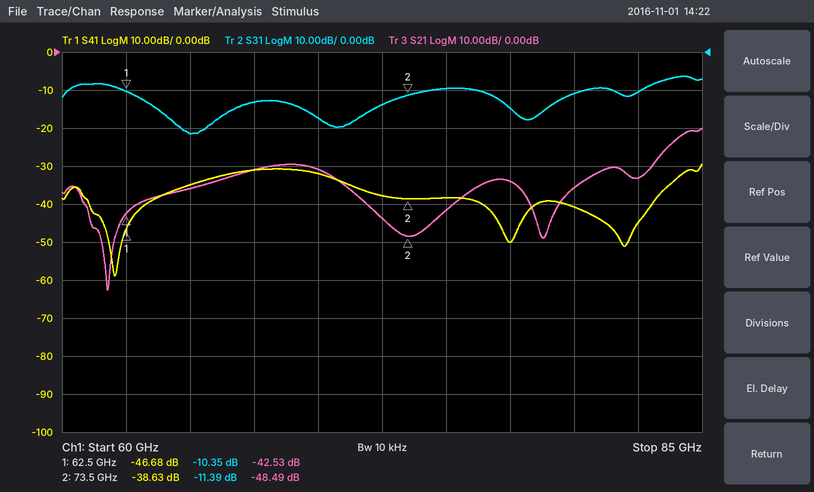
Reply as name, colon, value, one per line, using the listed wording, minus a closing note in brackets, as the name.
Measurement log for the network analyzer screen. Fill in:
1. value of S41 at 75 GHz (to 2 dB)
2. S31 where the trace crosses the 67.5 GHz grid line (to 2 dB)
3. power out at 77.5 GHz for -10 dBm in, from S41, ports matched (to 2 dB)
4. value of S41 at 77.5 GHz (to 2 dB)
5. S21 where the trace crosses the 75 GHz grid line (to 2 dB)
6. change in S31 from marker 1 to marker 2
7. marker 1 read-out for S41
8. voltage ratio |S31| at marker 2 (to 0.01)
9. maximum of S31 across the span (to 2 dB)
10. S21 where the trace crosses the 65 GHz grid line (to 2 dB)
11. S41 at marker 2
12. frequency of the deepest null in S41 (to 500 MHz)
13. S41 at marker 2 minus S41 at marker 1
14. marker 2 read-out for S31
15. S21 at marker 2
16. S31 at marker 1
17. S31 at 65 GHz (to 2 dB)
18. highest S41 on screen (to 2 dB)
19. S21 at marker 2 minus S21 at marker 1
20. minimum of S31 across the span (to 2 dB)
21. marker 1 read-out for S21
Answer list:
value of S41 at 75 GHz: -38 dB
S31 where the trace crosses the 67.5 GHz grid line: -14 dB
power out at 77.5 GHz for -10 dBm in, from S41, ports matched: -60 dBm
value of S41 at 77.5 GHz: -50 dB
S21 where the trace crosses the 75 GHz grid line: -42 dB
change in S31 from marker 1 to marker 2: -1.04 dB
marker 1 read-out for S41: -46.68 dB
voltage ratio |S31| at marker 2: 0.27
maximum of S31 across the span: -6 dB
S21 where the trace crosses the 65 GHz grid line: -36 dB
S41 at marker 2: -38.63 dB
frequency of the deepest null in S41: 62.0 GHz
S41 at marker 2 minus S41 at marker 1: 8.05 dB
marker 2 read-out for S31: -11.39 dB
S21 at marker 2: -48.49 dB
S31 at marker 1: -10.35 dB
S31 at 65 GHz: -22 dB
highest S41 on screen: -30 dB
S21 at marker 2 minus S21 at marker 1: -5.96 dB
minimum of S31 across the span: -22 dB
marker 1 read-out for S21: -42.53 dB
